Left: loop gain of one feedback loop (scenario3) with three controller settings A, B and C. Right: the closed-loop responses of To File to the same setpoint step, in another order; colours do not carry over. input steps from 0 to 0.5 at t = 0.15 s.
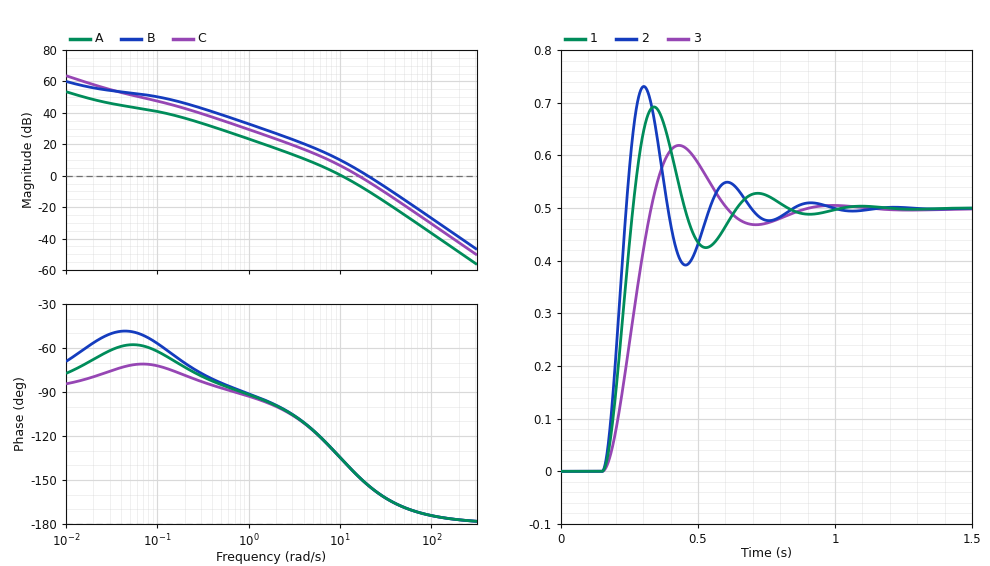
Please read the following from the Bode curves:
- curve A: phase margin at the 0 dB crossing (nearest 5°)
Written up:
45°
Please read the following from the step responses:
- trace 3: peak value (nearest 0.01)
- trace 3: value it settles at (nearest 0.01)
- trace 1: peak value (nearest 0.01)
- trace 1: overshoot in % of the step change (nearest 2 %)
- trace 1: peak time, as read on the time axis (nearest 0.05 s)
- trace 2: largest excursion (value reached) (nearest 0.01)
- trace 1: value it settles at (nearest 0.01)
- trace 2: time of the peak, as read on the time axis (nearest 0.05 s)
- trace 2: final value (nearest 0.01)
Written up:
0.62
0.50
0.69
38 %
0.35 s
0.73
0.50
0.30 s
0.50
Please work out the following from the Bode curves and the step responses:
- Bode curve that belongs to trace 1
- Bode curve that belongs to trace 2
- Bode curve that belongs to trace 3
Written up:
C
B
A
